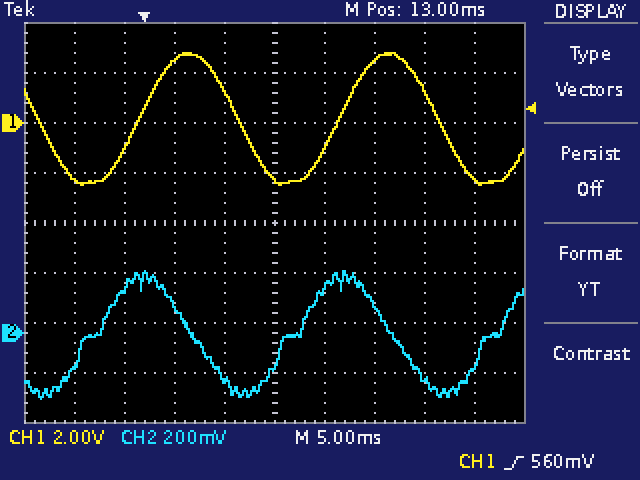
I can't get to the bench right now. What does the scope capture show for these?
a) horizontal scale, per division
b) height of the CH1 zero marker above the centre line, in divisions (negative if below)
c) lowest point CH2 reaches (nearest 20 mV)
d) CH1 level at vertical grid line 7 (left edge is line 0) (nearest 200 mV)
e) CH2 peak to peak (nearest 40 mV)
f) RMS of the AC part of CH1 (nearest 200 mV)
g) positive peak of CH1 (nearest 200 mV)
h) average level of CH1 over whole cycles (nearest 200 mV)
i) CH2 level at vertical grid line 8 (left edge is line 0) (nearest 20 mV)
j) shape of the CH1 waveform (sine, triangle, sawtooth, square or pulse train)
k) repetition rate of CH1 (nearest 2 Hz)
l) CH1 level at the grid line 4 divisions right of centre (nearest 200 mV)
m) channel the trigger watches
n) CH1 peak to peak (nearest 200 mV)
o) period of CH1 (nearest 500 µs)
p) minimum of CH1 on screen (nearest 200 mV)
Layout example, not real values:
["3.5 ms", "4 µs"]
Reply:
["5 ms", "+2.0 div", "-260 mV", "2.4 V", "520 mV", "1.8 V", "2.8 V", "200 mV", "-180 mV", "sine", "50 Hz", "-2.2 V", "CH1", "5.2 V", "20.0 ms", "-2.4 V"]
